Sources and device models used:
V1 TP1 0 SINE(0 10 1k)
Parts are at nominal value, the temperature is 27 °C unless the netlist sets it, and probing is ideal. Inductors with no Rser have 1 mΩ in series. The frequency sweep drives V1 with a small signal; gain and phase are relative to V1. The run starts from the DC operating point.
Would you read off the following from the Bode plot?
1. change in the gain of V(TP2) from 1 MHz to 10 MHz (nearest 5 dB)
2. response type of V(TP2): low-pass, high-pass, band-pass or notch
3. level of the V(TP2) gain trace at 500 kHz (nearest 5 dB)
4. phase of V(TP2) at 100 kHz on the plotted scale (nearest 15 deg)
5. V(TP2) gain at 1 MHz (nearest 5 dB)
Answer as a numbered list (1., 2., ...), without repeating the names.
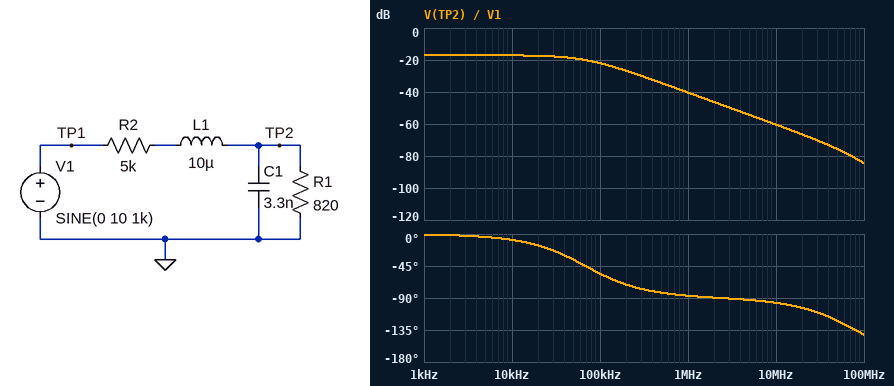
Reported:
1. -20 dB
2. low-pass
3. -35 dB
4. -60 deg
5. -40 dB
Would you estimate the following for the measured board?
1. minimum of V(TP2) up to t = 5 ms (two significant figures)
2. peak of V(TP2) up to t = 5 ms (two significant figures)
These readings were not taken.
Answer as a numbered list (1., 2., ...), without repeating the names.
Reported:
1. -1.4 V
2. 1.4 V
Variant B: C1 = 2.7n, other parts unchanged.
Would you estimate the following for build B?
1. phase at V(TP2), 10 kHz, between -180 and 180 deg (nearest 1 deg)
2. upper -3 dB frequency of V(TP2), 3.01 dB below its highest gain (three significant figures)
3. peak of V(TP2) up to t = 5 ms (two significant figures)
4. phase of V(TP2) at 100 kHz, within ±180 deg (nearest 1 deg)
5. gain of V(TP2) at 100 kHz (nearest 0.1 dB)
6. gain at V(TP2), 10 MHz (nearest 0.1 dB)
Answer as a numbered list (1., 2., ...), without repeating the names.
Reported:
1. -7 deg
2. 83.7 kHz
3. 1.4 V
4. -50 deg
5. -20.9 dB
6. -58.6 dB
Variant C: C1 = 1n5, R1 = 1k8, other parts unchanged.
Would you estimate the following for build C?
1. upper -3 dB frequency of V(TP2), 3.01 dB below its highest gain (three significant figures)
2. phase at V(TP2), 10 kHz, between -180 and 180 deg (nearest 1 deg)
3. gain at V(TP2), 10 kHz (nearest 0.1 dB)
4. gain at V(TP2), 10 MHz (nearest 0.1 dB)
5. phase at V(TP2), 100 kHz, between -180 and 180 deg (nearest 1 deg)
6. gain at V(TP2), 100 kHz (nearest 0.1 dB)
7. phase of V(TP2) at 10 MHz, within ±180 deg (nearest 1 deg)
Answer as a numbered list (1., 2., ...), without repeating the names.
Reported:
1. 80.2 kHz
2. -7 deg
3. -11.6 dB
4. -53.5 dB
5. -51 deg
6. -15.6 dB
7. -97 deg
